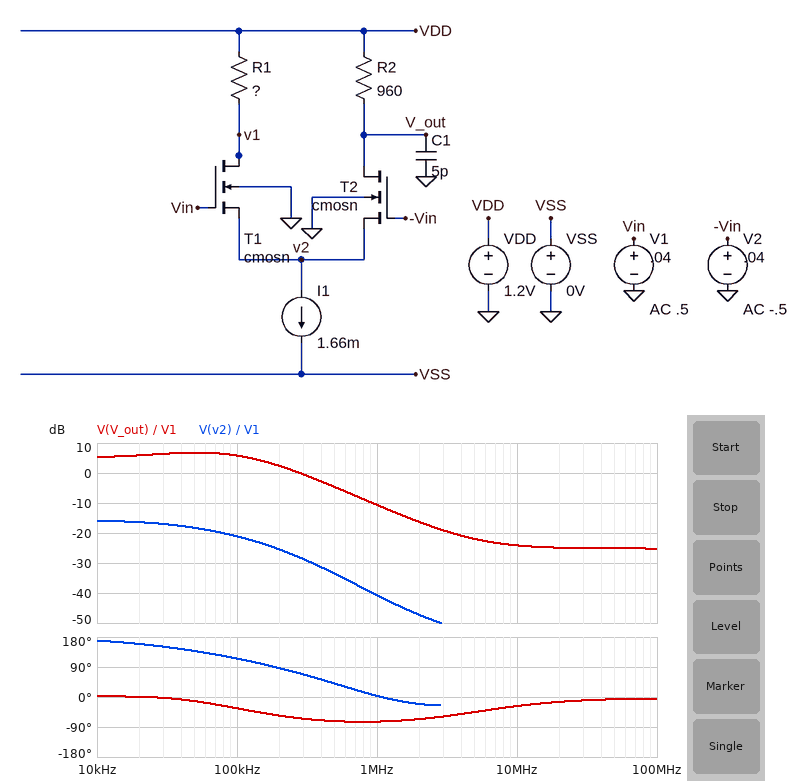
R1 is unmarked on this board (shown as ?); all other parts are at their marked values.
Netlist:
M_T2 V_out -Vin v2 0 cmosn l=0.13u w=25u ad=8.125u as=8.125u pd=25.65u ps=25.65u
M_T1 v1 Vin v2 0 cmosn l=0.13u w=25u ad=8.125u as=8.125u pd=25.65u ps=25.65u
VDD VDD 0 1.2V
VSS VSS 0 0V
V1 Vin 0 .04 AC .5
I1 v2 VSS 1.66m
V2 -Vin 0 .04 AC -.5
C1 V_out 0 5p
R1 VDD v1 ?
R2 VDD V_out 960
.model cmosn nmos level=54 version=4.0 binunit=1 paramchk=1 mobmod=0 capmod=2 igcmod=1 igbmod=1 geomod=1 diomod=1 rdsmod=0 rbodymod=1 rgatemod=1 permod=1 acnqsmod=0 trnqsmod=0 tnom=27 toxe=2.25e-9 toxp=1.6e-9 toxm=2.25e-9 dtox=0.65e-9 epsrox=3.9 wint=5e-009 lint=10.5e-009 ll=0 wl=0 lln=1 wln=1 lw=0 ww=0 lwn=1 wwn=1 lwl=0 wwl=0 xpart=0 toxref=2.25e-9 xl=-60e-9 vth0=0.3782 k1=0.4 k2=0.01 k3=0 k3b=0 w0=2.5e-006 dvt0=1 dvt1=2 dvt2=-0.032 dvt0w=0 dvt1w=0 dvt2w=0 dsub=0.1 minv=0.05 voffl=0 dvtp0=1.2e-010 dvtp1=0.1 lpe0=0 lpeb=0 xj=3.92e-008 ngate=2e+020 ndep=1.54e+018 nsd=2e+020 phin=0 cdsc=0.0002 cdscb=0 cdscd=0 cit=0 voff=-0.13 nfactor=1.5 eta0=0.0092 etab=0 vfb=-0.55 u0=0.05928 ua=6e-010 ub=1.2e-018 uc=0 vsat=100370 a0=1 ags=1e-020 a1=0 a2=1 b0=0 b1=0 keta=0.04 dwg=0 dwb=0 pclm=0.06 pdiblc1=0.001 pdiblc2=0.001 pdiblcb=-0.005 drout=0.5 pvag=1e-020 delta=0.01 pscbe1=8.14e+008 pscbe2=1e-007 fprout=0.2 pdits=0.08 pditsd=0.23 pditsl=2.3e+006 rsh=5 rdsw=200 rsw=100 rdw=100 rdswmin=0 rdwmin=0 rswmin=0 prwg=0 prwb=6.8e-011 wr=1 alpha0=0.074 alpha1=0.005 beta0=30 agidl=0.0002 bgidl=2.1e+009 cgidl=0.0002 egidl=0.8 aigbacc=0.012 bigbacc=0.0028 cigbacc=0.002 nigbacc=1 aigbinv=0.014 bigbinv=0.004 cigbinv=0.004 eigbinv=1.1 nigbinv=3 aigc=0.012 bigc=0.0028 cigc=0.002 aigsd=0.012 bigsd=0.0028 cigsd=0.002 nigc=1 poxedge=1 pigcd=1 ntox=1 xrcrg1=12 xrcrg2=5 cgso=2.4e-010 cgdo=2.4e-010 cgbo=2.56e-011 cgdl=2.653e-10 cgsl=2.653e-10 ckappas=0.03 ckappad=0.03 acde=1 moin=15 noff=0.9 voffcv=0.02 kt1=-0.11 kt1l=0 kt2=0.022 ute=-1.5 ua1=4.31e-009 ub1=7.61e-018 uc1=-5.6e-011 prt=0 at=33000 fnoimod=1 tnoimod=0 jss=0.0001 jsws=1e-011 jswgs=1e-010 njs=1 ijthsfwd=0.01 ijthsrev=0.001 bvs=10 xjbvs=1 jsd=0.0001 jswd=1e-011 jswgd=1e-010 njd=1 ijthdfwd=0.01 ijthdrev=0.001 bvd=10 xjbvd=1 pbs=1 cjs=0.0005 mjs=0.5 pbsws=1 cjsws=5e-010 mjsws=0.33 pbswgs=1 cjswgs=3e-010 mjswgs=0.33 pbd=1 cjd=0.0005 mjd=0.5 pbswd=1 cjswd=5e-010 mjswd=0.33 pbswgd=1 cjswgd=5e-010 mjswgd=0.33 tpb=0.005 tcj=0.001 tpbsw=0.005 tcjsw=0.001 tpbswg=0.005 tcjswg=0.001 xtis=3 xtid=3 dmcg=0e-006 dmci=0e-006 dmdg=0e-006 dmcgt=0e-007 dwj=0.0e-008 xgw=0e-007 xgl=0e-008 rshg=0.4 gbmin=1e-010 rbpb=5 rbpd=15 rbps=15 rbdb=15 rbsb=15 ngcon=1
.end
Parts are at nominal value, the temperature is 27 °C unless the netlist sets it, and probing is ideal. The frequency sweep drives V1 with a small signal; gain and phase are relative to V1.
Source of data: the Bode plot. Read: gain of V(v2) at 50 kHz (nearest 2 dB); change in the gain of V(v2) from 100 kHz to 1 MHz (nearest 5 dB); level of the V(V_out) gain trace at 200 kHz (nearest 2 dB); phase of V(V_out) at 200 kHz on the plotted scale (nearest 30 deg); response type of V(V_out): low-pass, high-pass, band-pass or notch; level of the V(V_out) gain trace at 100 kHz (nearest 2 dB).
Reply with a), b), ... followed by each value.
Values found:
a) -18 dB
b) -20 dB
c) 2 dB
d) -60 deg
e) low-pass
f) 6 dB
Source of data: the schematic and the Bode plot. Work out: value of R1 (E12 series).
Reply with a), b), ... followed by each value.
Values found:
a) 2.7 kΩ
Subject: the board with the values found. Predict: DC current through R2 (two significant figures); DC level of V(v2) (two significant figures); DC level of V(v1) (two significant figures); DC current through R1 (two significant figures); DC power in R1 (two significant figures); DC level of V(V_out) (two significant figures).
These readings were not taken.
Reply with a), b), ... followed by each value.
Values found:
a) 1.0 mA
b) -290 mV
c) -220 mV
d) 530 µA
e) 750 µW
f) 210 mV
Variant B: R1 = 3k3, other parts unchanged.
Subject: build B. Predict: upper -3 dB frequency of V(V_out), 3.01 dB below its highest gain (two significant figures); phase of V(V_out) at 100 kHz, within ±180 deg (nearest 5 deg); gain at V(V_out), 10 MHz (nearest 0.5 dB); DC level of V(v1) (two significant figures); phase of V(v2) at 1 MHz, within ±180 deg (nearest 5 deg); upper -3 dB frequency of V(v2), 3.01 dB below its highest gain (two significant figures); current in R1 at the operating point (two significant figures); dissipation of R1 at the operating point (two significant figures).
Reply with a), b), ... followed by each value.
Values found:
a) 180 kHz
b) -30 deg
c) -24.0 dB
d) -250 mV
e) 105 deg
f) 170 kHz
g) 440 µA
h) 640 µW
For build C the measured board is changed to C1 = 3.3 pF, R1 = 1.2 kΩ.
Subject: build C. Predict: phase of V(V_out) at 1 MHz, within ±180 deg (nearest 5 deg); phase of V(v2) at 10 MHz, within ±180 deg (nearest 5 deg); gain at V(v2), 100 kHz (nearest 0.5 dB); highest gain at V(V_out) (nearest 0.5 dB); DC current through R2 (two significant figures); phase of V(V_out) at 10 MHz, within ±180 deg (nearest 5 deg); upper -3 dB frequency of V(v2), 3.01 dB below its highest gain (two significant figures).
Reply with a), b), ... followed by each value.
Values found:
a) -80 deg
b) -20 deg
c) -16.5 dB
d) 12.0 dB
e) 850 µA
f) -30 deg
g) 490 kHz
